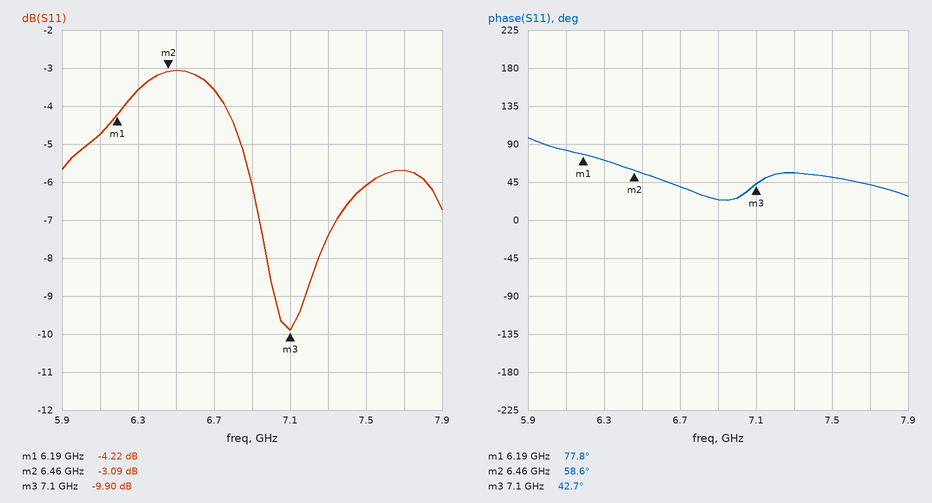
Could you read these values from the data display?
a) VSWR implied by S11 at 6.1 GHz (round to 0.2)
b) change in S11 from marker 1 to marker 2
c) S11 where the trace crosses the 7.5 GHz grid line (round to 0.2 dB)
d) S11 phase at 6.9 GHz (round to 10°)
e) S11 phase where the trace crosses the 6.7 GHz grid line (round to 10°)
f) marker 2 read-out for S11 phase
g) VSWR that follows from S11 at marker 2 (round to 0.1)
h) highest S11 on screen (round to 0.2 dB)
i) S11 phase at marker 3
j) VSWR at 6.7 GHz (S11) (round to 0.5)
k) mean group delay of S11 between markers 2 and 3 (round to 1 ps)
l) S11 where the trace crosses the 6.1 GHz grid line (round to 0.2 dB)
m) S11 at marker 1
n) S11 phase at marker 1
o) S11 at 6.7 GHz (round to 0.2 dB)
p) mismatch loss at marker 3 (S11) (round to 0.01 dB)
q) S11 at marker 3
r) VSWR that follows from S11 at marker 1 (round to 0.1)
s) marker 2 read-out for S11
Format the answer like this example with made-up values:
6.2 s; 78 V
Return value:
3.8; 1.13 dB; -6.0 dB; 20°; 40°; 58.6°; 5.7; -3.0 dB; 42.7°; 5.0; 69 ps; -4.8 dB; -4.22 dB; 77.8°; -3.6 dB; 0.47 dB; -9.90 dB; 4.2; -3.09 dB
